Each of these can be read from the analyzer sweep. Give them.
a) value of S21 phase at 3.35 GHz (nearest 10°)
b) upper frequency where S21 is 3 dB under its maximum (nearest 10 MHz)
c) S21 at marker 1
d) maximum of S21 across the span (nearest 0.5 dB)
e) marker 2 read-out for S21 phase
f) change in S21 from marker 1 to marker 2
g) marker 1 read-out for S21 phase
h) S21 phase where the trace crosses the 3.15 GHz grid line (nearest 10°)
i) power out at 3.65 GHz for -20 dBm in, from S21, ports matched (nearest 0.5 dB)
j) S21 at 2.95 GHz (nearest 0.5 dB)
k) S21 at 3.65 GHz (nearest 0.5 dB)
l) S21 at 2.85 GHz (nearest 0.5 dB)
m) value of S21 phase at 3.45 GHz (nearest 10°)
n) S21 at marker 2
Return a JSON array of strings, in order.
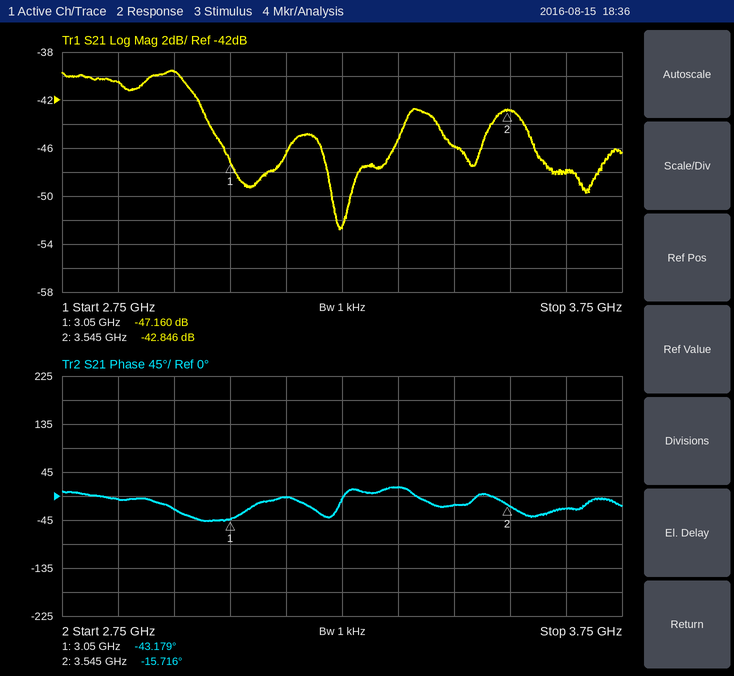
["20°", "3.00 GHz", "-47.160 dB", "-39.5 dB", "-15.716°", "4.314 dB", "-43.179°", "0°", "-68.0 dBm", "-39.5 dB", "-48.0 dB", "-40.5 dB", "-20°", "-42.846 dB"]
